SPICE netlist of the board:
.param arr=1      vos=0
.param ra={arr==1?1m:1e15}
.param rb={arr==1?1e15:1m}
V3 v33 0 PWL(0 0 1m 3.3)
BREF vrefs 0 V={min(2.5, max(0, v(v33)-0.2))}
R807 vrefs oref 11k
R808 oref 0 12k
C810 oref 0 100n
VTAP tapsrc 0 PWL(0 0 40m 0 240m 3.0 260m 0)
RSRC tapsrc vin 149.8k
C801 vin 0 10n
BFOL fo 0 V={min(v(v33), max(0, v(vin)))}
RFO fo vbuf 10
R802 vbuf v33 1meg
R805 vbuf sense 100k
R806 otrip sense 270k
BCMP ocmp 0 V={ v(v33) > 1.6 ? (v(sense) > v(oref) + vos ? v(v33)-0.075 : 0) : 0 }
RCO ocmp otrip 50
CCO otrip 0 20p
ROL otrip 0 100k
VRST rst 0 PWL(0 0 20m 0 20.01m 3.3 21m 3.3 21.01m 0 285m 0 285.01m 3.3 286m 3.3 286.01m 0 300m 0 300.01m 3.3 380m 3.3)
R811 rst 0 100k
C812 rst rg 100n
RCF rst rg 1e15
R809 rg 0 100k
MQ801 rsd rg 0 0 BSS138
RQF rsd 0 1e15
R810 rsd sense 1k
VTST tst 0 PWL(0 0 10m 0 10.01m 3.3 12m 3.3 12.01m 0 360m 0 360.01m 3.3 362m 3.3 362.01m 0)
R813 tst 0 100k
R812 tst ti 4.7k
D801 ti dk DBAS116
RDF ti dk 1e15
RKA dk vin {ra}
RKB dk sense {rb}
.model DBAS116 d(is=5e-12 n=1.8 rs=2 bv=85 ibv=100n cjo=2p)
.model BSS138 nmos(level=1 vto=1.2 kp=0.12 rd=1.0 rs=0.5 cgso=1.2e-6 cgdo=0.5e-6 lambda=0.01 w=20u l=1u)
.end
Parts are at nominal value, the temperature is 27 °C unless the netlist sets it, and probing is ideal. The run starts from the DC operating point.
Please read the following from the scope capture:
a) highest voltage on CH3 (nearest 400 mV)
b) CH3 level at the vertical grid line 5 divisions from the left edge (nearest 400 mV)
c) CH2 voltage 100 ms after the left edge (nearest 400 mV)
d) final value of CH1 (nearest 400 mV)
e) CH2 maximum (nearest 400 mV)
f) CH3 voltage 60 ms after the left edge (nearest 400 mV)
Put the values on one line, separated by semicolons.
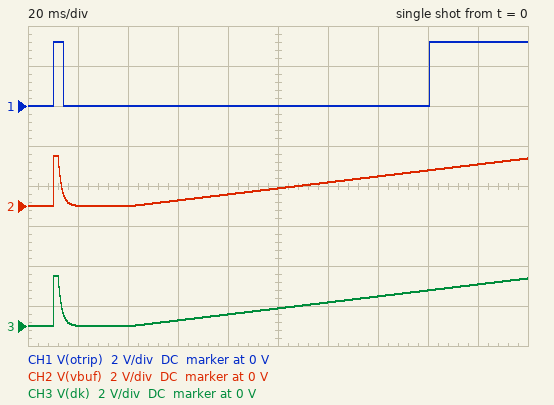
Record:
2.4 V; 800 mV; 800 mV; 3.2 V; 2.4 V; 400 mV
